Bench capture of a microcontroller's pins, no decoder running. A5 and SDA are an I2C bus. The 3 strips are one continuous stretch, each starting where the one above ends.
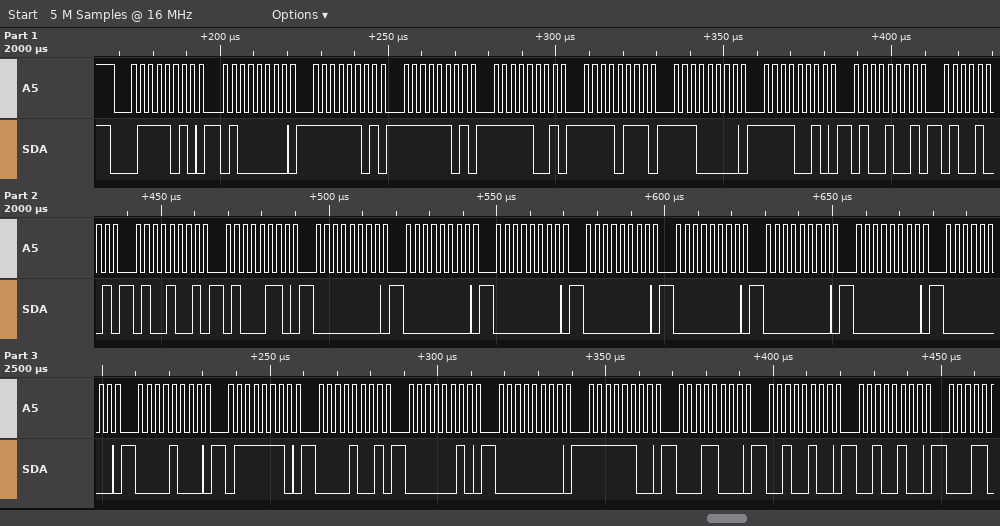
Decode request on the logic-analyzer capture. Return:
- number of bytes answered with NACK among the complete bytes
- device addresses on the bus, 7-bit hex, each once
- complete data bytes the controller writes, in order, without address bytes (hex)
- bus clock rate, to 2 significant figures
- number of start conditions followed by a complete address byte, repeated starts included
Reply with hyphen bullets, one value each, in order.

- 0
- 0x3D
- 40 FD FD F9 F7 E0 F2 49 49 49 46 00 00 00 00 00 00 00 00 08 7E 09 02 00 FC 18 24 24
- 400 kHz
- 1
